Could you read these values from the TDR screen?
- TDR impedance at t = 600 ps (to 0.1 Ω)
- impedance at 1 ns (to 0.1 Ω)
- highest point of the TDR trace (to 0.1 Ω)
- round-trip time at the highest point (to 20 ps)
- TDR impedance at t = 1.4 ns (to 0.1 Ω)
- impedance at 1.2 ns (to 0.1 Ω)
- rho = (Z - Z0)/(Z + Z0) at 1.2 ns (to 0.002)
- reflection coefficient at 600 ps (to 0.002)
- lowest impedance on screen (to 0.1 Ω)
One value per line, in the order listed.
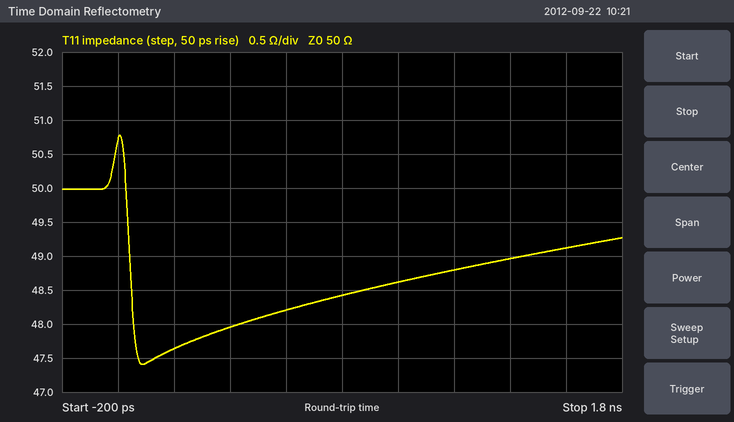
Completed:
48.2 Ω
48.6 Ω
50.8 Ω
0 ps
49.0 Ω
48.8 Ω
-0.012
-0.018
47.4 Ω
